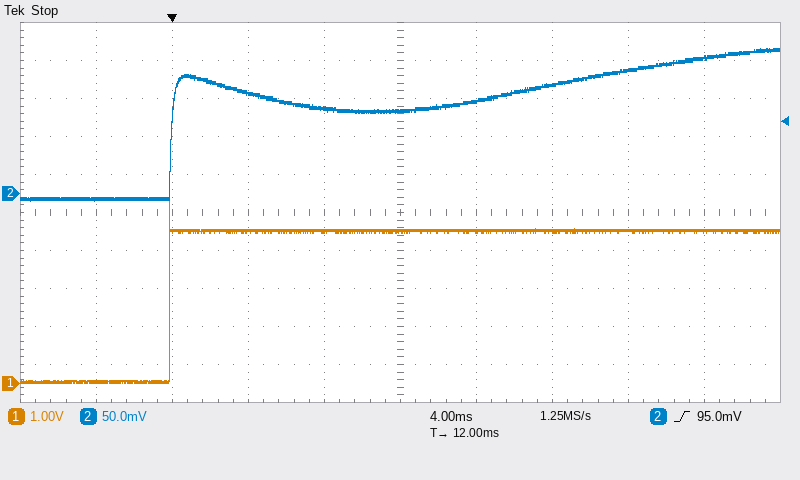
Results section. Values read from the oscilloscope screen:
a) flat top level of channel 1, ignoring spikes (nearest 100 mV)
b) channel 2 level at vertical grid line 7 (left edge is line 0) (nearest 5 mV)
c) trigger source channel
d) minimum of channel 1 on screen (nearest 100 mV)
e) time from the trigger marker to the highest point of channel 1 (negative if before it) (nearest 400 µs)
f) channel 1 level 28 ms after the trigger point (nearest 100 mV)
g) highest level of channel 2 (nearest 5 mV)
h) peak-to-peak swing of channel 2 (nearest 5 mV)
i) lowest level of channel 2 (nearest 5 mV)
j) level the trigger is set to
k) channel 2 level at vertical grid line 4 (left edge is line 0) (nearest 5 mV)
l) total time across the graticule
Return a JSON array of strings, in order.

["4.0 V", "140 mV", "channel 2", "0.0 V", "0.0 ms", "4.0 V", "190 mV", "200 mV", "-10 mV", "95.0 mV", "110 mV", "40 ms"]
